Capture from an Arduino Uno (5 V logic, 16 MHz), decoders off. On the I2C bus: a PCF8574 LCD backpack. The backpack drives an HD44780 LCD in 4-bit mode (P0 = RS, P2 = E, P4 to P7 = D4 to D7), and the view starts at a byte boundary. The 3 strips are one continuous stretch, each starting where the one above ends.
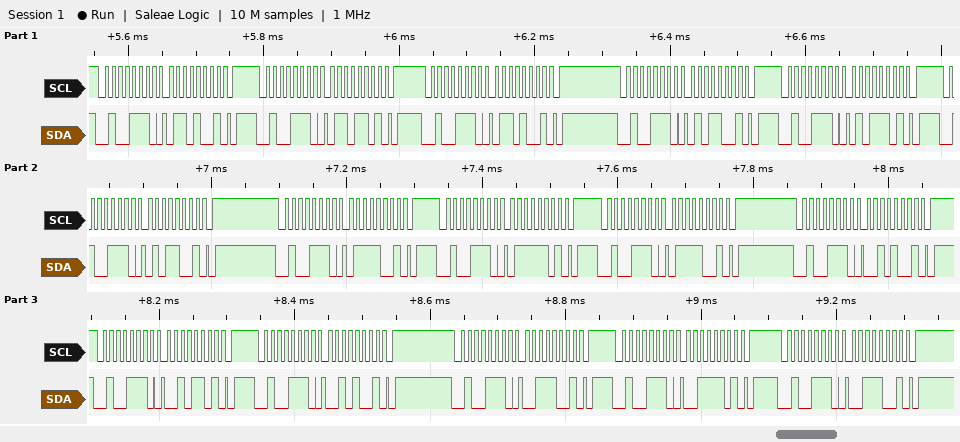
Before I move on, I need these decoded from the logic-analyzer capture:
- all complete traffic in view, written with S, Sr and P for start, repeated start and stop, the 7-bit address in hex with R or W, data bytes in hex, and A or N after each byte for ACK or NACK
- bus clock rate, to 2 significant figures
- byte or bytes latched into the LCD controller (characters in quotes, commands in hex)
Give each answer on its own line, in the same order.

S 27W A 69 A P S 27W A 6D A P S 27W A 69 A P S 27W A 59 A P S 27W A 5D A P S 27W A 59 A P S 27W A 79 A P S 27W A 7D A P S 27W A 79 A P S 27W A 29 A P S 27W A 2D A P S 27W A 29 A P S 27W A 39 A P S 27W A 3D A P S 27W A 39 A P
100 kHz
'e' 'r'
